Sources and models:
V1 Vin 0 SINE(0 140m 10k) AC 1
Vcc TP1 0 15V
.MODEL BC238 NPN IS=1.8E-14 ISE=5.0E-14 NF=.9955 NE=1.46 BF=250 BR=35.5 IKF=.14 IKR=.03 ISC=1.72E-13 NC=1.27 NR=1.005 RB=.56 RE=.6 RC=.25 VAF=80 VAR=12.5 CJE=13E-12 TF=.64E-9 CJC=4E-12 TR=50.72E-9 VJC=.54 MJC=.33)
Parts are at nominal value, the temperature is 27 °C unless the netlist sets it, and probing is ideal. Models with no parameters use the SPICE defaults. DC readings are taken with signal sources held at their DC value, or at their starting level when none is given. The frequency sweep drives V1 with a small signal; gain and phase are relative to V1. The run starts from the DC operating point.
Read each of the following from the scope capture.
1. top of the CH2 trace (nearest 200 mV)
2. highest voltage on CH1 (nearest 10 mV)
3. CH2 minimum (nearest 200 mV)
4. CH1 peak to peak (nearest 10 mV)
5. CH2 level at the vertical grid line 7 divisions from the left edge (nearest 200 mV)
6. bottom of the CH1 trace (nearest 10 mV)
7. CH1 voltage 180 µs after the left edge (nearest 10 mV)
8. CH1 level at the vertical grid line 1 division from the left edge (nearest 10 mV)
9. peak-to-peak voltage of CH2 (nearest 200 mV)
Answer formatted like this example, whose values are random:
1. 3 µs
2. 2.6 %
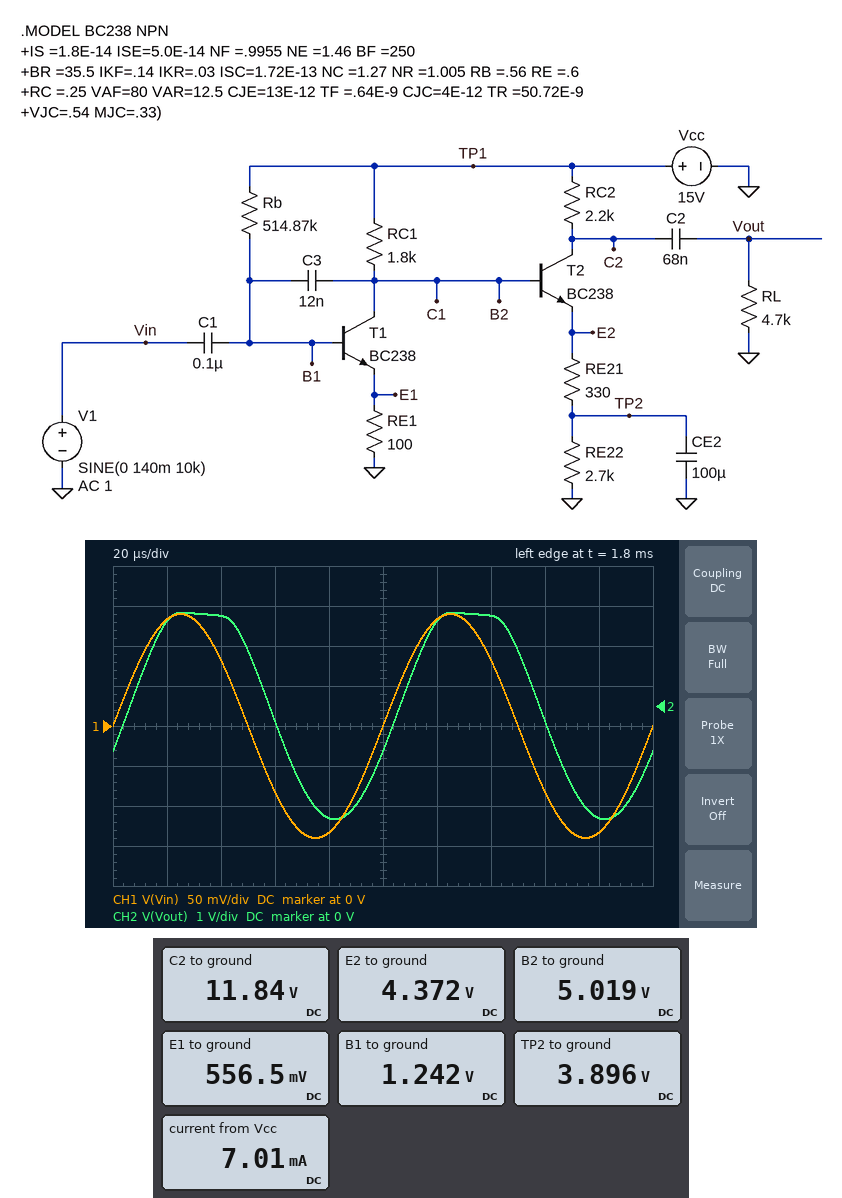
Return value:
1. 2.4 V
2. 140 mV
3. -2.8 V
4. 280 mV
5. 2.2 V
6. -140 mV
7. -130 mV
8. 130 mV
9. 5.2 V
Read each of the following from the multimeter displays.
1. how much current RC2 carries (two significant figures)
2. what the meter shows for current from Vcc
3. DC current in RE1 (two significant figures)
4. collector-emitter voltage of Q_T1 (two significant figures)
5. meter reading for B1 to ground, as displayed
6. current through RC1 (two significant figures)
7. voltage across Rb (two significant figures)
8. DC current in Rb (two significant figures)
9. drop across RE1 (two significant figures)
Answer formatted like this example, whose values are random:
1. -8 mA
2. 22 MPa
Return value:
1. 1.4 mA
2. 7.01 mA
3. 5.6 mA
4. 4.5 V
5. 1.242 V
6. 5.5 mA
7. 14 V
8. 27 µA
9. 560 mV
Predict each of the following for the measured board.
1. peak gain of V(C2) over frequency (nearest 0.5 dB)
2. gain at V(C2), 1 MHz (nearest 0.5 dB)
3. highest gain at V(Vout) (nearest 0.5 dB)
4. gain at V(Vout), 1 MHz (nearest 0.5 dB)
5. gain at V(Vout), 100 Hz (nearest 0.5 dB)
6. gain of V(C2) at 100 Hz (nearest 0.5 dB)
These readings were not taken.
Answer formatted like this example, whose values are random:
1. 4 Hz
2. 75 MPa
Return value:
1. 30.0 dB
2. 12.5 dB
3. 27.0 dB
4. 12.5 dB
5. 16.0 dB
6. 30.0 dB
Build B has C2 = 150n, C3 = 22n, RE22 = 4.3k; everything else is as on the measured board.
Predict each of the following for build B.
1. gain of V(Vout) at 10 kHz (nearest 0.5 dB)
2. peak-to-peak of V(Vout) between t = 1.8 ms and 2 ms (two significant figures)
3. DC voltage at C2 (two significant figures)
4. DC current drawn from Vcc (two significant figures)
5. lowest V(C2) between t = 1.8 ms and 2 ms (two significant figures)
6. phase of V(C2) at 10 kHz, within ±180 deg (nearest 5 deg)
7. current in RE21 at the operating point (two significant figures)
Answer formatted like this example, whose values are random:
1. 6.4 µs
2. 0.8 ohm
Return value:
1. 22.0 dB
2. 3.2 V
3. 13 V
4. 6.5 mA
5. 11 V
6. -35 deg
7. 950 µA
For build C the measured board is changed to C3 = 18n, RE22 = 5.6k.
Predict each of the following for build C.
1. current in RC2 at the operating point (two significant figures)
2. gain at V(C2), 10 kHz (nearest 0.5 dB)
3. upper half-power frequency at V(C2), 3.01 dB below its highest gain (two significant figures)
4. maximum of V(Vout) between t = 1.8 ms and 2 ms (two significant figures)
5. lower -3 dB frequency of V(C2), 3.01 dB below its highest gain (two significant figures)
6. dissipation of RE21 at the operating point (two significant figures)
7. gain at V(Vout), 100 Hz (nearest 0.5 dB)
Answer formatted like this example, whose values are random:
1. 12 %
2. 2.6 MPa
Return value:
1. 740 µA
2. 23.5 dB
3. 3.4 kHz
4. 1.4 V
5. 20 Hz
6. 180 µW
7. 13.0 dB
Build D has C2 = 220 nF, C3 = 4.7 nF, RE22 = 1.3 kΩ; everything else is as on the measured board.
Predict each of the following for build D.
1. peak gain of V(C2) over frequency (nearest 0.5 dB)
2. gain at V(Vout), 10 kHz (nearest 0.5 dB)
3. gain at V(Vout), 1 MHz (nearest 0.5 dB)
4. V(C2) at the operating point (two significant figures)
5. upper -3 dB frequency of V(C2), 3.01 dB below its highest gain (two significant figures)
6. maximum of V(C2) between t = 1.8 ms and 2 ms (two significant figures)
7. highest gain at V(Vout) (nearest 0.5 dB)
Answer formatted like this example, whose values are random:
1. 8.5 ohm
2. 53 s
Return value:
1. 33.0 dB
2. 31.5 dB
3. 13.0 dB
4. 9.2 V
5. 26 kHz
6. 13 V
7. 32.0 dB
